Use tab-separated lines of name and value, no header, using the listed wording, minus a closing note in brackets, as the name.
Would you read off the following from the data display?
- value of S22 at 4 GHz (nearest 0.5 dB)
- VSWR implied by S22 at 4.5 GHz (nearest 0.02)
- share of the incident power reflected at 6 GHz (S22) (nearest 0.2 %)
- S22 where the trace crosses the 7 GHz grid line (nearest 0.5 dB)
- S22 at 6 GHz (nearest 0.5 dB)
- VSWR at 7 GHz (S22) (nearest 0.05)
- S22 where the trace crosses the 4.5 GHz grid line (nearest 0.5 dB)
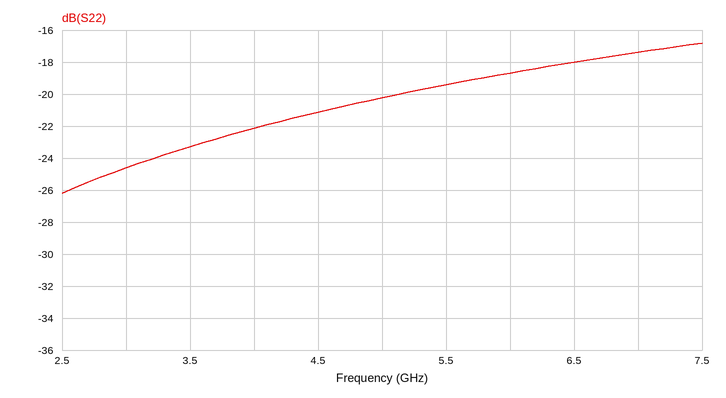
value of S22 at 4 GHz	-22.0 dB
VSWR implied by S22 at 4.5 GHz	1.20
share of the incident power reflected at 6 GHz (S22)	1.4 %
S22 where the trace crosses the 7 GHz grid line	-17.5 dB
S22 at 6 GHz	-18.5 dB
VSWR at 7 GHz (S22)	1.30
S22 where the trace crosses the 4.5 GHz grid line	-21.0 dB
